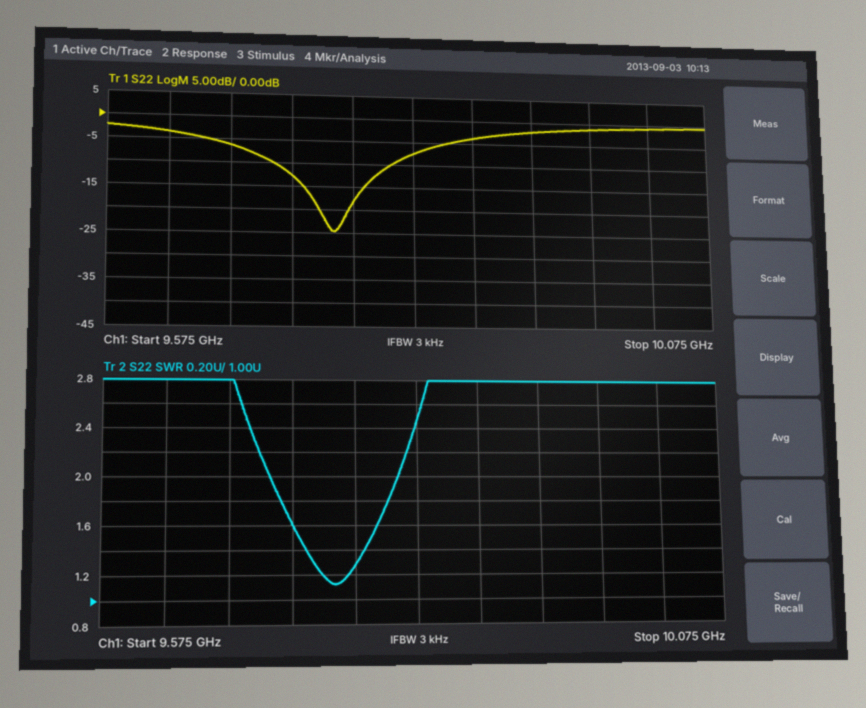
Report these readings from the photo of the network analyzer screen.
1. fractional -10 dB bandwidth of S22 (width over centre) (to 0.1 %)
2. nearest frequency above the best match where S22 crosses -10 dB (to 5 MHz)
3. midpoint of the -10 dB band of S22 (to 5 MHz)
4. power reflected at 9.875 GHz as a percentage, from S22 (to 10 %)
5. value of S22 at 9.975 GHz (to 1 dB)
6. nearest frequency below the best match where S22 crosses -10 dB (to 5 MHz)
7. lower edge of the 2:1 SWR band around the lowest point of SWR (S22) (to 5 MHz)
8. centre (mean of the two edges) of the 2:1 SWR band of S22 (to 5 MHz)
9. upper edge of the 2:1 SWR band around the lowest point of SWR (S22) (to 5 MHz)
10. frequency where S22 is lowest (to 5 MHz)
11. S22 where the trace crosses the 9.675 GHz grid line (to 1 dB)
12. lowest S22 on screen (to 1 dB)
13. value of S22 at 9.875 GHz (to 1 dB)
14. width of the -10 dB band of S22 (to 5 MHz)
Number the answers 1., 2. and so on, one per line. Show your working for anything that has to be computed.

1. 95 MHz / 9.7575 GHz ≈ 1.0 %
2. 9.805 GHz
3. 9.760 GHz
4. 10^(-4/10) ≈ 40 %
5. -1 dB
6. 9.710 GHz
7. 9.705 GHz
8. 9.760 GHz
9. 9.810 GHz
10. 9.760 GHz
11. -6 dB
12. -25 dB
13. -4 dB
14. 9.805 GHz − 9.710 GHz = 95 MHz
